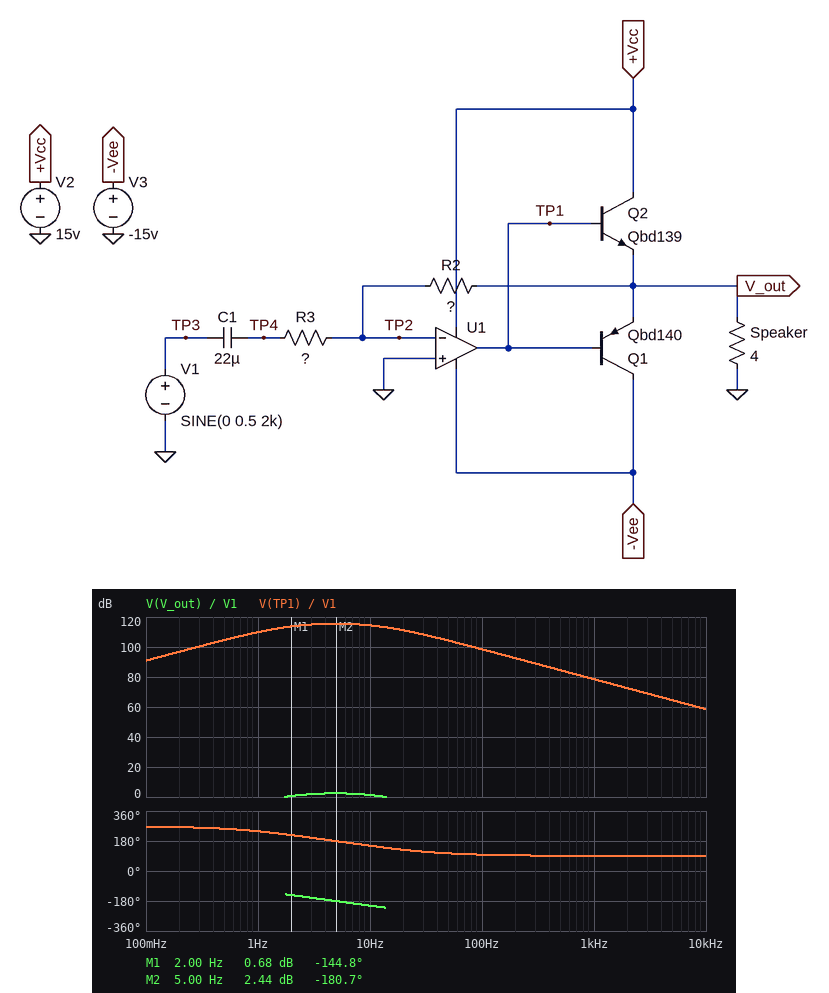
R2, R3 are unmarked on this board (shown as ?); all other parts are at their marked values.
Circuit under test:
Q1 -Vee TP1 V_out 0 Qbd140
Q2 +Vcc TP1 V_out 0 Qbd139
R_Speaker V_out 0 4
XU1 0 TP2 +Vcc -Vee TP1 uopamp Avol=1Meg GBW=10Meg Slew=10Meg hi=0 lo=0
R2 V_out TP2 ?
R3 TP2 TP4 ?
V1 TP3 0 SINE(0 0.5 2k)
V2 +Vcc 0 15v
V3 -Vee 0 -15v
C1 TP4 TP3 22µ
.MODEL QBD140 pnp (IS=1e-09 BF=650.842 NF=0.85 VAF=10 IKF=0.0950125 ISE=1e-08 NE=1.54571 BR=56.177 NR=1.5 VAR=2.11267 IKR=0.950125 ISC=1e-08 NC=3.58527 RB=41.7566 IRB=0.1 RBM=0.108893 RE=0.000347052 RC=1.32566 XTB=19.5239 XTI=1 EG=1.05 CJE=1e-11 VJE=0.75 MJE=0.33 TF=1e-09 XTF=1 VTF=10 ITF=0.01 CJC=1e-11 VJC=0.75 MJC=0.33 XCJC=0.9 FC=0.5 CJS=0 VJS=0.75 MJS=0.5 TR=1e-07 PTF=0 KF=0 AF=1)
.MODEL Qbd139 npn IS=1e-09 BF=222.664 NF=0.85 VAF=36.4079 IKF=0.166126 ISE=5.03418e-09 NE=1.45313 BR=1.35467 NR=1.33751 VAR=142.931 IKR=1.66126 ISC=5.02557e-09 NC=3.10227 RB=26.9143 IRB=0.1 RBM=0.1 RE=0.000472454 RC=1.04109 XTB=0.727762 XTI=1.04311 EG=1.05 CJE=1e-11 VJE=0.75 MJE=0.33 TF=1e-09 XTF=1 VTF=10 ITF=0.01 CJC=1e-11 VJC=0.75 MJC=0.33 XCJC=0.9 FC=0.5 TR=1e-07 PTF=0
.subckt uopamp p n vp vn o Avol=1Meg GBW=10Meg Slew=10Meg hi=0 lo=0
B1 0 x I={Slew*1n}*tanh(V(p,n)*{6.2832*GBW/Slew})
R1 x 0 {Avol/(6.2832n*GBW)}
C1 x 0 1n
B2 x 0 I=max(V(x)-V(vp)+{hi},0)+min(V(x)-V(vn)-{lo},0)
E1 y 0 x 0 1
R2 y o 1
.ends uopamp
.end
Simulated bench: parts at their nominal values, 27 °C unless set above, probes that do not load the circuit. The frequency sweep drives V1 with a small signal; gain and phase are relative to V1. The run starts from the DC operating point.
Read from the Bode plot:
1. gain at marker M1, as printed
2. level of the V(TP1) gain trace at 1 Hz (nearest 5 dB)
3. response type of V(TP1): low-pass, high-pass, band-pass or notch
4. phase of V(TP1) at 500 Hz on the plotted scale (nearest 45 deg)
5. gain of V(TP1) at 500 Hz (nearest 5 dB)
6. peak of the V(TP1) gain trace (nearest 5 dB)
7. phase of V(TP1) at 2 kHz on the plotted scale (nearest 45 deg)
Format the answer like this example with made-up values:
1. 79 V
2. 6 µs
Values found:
1. 0.68 dB
2. 110 dB
3. band-pass
4. 90 deg
5. 85 dB
6. 115 dB
7. 90 deg
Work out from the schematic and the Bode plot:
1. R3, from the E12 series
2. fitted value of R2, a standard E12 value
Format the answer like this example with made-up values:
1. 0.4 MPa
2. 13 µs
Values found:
1. 1.5 kΩ
2. 8.2 kΩ
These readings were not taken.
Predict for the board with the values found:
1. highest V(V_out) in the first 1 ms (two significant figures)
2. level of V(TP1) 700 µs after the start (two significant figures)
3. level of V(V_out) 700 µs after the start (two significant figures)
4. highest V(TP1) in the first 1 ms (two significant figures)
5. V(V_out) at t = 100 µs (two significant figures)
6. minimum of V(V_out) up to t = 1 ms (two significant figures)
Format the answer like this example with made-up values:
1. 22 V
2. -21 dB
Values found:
1. 2.7 V
2. -2.1 V
3. -1.6 V
4. 3.5 V
5. -2.6 V
6. -2.7 V
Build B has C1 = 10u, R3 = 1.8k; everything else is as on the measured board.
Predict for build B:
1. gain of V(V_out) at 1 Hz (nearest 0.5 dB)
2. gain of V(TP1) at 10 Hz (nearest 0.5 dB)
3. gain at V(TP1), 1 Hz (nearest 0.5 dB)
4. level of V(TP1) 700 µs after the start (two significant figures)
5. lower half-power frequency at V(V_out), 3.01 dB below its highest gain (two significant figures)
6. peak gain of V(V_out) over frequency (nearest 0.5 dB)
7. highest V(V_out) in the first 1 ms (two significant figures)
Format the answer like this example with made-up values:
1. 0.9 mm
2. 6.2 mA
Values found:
1. -9.0 dB
2. 114.0 dB
3. 104.0 dB
4. -1.8 V
5. 2.8 Hz
6. 1.5 dB
7. 2.3 V
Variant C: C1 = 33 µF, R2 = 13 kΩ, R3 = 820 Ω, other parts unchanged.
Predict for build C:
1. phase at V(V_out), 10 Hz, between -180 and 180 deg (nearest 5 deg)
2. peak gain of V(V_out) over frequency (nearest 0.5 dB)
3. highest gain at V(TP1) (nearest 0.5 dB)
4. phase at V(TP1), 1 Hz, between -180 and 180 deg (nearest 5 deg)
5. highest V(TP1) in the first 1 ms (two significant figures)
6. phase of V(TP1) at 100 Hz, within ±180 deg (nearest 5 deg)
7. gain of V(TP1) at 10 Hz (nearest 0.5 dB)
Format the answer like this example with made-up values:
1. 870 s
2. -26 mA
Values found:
1. 145 deg
2. 5.0 dB
3. 118.0 dB
4. -140 deg
5. 9.7 V
6. 95 deg
7. 116.0 dB
